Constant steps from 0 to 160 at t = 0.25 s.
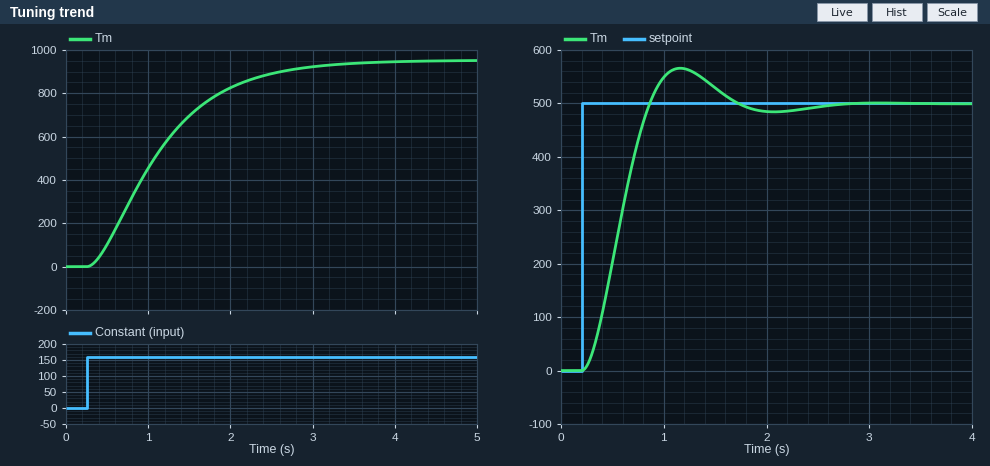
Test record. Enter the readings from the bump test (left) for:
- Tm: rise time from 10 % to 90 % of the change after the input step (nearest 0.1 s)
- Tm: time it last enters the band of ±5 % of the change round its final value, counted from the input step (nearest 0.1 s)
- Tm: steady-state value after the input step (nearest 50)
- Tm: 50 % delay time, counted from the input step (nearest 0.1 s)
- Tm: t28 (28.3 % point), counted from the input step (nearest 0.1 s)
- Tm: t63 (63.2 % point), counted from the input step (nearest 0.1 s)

1.7 s
2.4 s
950
0.8 s
0.5 s
1.0 s
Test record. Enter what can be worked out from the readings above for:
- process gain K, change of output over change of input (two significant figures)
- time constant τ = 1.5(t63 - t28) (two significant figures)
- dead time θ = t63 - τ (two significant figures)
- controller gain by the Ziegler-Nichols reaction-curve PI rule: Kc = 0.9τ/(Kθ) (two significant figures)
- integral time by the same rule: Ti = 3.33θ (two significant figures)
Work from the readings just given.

5.9
0.75 s
0.25 s
0.46
0.83 s
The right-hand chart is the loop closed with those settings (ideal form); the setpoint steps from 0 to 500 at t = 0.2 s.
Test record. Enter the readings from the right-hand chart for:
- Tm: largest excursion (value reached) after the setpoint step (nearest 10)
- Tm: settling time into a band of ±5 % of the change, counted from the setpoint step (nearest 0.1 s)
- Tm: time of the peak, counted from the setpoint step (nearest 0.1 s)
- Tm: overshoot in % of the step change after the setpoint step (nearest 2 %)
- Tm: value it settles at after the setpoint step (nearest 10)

570
1.3 s
1.0 s
14 %
500
